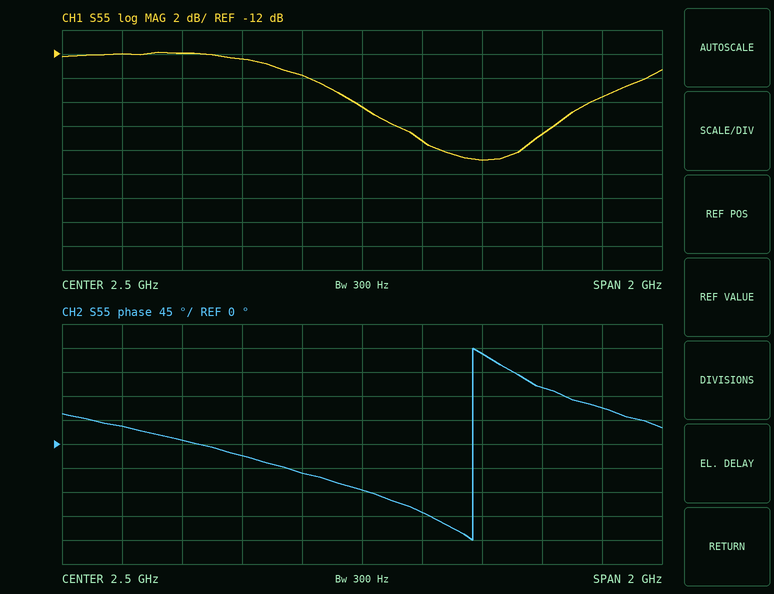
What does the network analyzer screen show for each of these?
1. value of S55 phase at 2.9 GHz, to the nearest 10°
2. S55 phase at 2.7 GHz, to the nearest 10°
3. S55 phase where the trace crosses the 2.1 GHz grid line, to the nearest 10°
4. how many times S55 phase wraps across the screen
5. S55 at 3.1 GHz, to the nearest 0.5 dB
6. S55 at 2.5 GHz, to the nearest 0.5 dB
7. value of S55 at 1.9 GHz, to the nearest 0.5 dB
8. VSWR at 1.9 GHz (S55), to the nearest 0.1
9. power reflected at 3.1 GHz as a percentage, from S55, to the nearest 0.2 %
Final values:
170°
-130°
-20°
1
-18.5 dB
-16.5 dB
-12.0 dB
1.7
1.4 %
